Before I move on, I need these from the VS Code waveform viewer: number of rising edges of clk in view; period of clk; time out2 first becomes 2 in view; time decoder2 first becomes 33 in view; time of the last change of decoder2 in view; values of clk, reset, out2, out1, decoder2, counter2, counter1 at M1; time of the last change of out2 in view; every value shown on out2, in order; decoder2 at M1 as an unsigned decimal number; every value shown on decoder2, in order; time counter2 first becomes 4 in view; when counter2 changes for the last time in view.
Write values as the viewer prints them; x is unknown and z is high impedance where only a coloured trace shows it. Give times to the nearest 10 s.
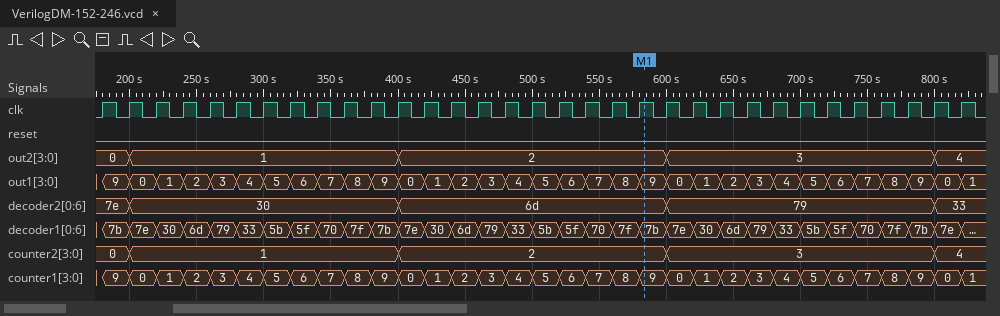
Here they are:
33
20 s
400 s
800 s
800 s
clk=1, reset=0, out2=2, out1=9, decoder2=6d, counter2=2, counter1=9
800 s
0, 1, 2, 3, 4
109
7e, 30, 6d, 79, 33
800 s
800 s
